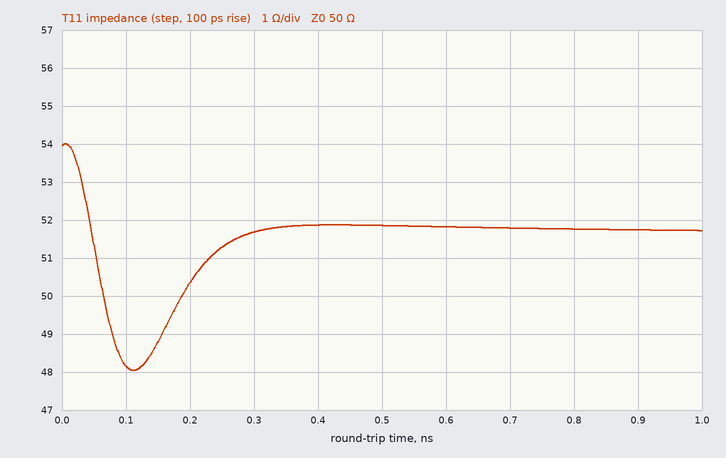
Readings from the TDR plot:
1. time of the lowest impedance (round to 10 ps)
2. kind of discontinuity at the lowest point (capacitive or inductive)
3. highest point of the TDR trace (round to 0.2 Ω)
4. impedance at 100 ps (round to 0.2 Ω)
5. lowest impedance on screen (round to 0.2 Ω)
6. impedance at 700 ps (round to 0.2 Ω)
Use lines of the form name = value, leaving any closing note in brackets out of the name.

time of the lowest impedance = 110 ps
kind of discontinuity at the lowest point = capacitive
highest point of the TDR trace = 54.0 Ω
impedance at 100 ps = 48.2 Ω
lowest impedance on screen = 48.0 Ω
impedance at 700 ps = 51.8 Ω
